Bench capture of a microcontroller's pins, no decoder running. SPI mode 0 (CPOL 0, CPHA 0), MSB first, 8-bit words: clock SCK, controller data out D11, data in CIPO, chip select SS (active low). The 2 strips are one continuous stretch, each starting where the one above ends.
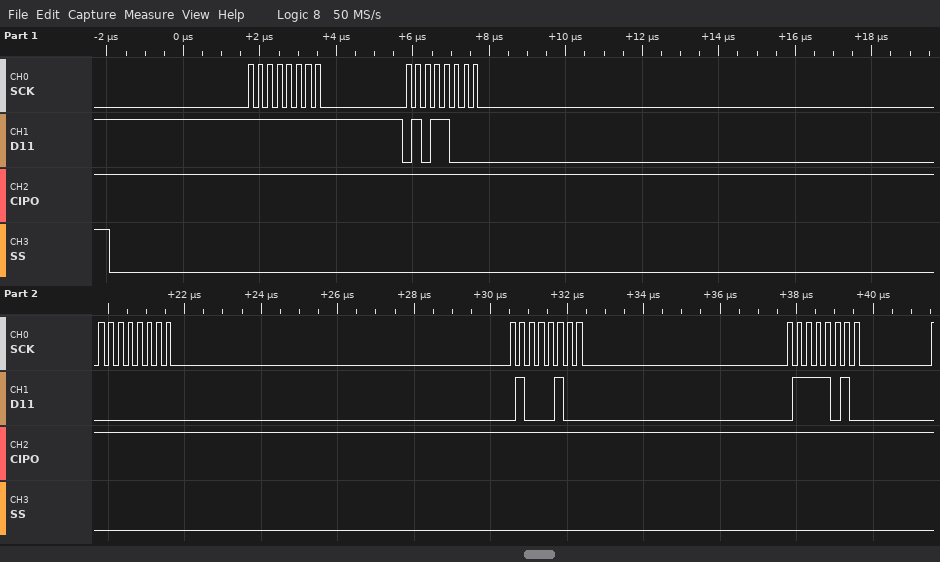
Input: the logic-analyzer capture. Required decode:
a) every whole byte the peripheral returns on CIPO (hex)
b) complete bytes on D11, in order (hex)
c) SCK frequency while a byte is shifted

FF FF FF FF FF
FF 58 00 44 7A
4 MHz
